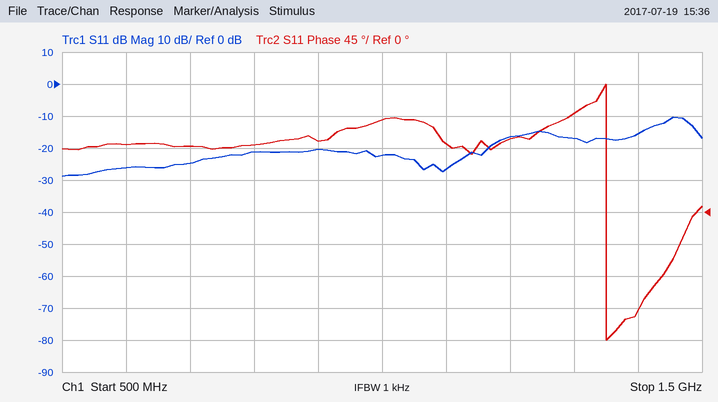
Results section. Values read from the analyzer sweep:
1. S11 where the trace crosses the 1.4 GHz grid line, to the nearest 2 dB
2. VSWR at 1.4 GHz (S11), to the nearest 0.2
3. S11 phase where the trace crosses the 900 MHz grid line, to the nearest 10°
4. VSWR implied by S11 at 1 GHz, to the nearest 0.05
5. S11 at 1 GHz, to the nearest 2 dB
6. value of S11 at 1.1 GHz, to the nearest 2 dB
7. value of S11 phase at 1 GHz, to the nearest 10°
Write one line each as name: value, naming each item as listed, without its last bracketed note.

S11 where the trace crosses the 1.4 GHz grid line, to the nearest 2 dB: -16 dB
VSWR at 1.4 GHz (S11), to the nearest 0.2: 1.4
S11 phase where the trace crosses the 900 MHz grid line, to the nearest 10°: 100°
VSWR implied by S11 at 1 GHz, to the nearest 0.05: 1.15
S11 at 1 GHz, to the nearest 2 dB: -22 dB
value of S11 at 1.1 GHz, to the nearest 2 dB: -26 dB
value of S11 phase at 1 GHz, to the nearest 10°: 130°
